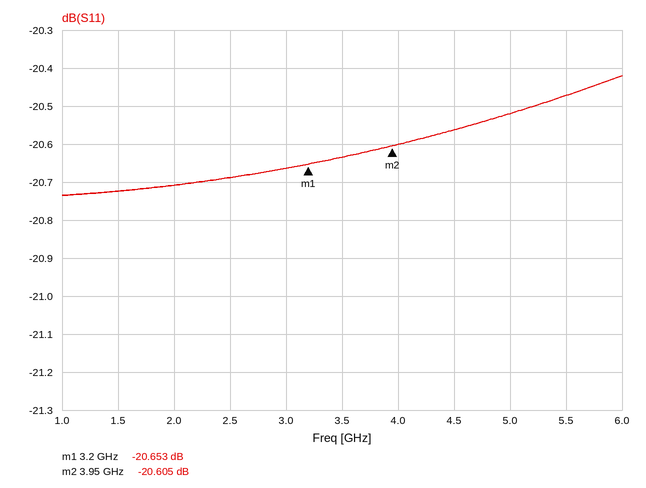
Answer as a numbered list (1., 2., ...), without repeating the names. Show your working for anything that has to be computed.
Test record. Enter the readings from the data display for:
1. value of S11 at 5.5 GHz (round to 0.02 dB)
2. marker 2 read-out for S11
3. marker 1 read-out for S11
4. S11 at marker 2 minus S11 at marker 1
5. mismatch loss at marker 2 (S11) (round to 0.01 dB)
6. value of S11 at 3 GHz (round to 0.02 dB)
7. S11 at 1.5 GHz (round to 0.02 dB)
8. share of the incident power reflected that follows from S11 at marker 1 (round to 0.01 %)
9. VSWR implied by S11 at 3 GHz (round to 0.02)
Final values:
1. -20.48 dB
2. -20.605 dB
3. -20.653 dB
4. -20.605 − (-20.653) = 0.048 dB
5. −10 log10(1 − 10^(-20.605/10)) ≈ 0.04 dB
6. -20.66 dB
7. -20.72 dB
8. 10^(-20.653/10) ≈ 0.86 %
9. |Γ| = 10^(-20.66/20) = 0.0927; VSWR = (1 + 0.0927)/(1 − 0.0927) ≈ 1.20
